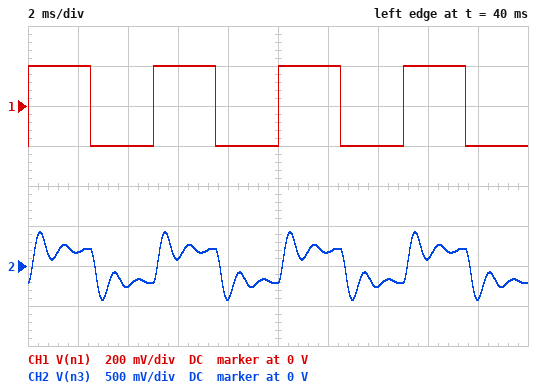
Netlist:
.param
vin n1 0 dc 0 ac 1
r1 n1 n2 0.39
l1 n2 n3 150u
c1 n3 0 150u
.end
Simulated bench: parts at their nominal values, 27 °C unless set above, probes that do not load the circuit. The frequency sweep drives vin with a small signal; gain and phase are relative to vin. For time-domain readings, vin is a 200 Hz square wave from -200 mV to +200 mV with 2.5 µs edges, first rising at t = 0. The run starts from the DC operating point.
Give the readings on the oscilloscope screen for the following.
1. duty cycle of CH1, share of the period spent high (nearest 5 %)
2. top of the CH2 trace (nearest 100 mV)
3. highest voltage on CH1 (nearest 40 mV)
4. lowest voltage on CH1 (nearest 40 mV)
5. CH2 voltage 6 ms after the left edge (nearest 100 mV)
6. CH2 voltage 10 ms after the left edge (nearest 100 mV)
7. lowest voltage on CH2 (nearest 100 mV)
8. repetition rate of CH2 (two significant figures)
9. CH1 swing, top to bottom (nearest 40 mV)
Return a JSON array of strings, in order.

["50 %", "400 mV", "200 mV", "-200 mV", "100 mV", "-200 mV", "-400 mV", "200 Hz", "400 mV"]
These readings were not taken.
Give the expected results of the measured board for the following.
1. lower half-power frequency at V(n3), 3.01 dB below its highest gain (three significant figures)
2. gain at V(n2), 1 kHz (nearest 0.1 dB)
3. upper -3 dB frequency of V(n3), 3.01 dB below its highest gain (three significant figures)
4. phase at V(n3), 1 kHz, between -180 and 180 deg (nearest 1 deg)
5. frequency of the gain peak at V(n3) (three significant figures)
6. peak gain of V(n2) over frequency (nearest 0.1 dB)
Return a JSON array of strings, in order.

["781 Hz", "-10.7 dB", "1.21 kHz", "-73 deg", "1.02 kHz", "0 dB"]
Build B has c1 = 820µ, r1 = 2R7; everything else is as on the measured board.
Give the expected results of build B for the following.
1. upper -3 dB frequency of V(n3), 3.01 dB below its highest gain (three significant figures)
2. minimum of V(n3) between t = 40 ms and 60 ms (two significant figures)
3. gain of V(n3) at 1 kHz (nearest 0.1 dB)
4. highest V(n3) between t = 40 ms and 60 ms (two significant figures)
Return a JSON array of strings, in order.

["73.7 Hz", "-100 mV", "-23.2 dB", "100 mV"]
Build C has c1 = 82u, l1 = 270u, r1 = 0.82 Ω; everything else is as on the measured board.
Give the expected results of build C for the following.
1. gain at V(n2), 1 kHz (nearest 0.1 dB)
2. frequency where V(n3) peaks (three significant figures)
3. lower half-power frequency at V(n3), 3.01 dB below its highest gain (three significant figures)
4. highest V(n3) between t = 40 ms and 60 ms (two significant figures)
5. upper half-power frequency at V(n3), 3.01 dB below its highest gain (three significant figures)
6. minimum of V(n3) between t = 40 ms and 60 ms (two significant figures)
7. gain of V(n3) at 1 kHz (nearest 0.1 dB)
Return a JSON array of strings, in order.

["-10.9 dB", "1.01 kHz", "724 Hz", "400 mV", "1.24 kHz", "-400 mV", "7.1 dB"]
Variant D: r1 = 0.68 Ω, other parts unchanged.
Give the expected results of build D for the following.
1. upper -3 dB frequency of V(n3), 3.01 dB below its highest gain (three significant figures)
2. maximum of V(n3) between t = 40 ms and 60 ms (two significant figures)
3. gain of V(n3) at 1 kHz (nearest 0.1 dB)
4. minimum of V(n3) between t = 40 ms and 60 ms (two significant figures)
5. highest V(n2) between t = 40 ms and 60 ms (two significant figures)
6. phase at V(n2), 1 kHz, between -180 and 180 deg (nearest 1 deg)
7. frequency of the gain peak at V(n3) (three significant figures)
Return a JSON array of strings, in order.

["1.26 kHz", "330 mV", "3.7 dB", "-330 mV", "260 mV", "-80 deg", "930 Hz"]
